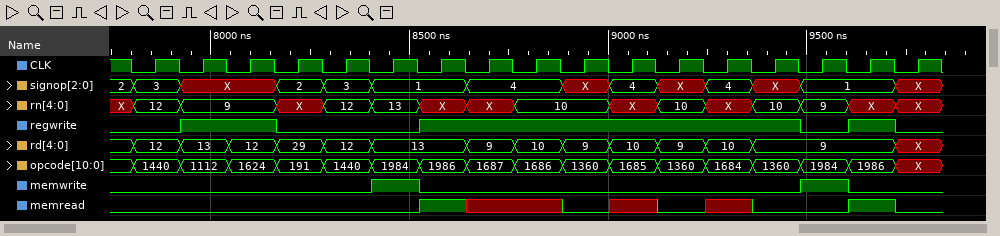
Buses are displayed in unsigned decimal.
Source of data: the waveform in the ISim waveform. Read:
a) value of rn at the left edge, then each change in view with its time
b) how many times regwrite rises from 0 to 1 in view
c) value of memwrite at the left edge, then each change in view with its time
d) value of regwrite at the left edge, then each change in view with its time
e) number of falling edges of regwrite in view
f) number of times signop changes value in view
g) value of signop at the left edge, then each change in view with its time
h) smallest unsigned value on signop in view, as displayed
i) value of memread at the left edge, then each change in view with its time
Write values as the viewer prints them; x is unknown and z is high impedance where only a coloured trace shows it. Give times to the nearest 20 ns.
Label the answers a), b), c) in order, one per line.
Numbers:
a) X, 12 at 7800 ns, 9 at 7920 ns, X at 8160 ns, 12 at 8280 ns, 13 at 8400 ns, X at 8520 ns, X at 8640 ns, 10 at 8760 ns, X at 9000 ns, 10 at 9120 ns, X at 9240 ns, 10 at 9360 ns, 9 at 9480 ns, X at 9600 ns, X at 9720 ns
b) 3
c) 0, 1 at 8400 ns, 0 at 8520 ns, 1 at 9480 ns, 0 at 9600 ns
d) 0, 1 at 7920 ns, 0 at 8160 ns, 1 at 8520 ns, 0 at 9480 ns, 1 at 9600 ns, 0 at 9720 ns
e) 3
f) 13
g) 2, 3 at 7800 ns, X at 7920 ns, 2 at 8160 ns, 3 at 8280 ns, 1 at 8400 ns, 4 at 8640 ns, X at 8880 ns, 4 at 9000 ns, X at 9120 ns, 4 at 9240 ns, X at 9360 ns, 1 at 9480 ns, X at 9720 ns
h) 1
i) 0, 1 at 8520 ns, x at 8640 ns, 0 at 8880 ns, x at 9000 ns, 0 at 9120 ns, x at 9240 ns, 0 at 9360 ns, 1 at 9600 ns, 0 at 9720 ns
